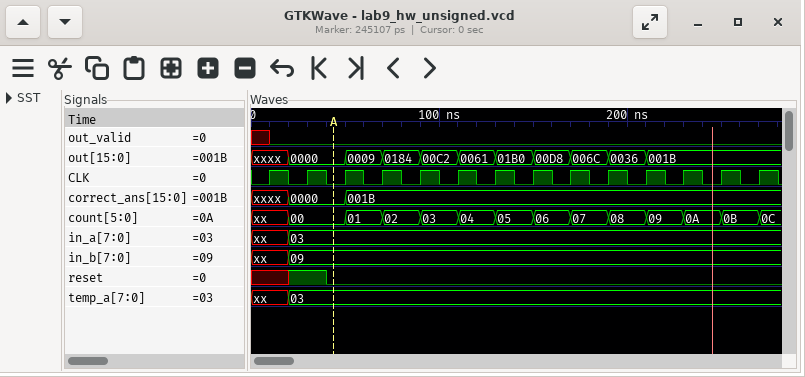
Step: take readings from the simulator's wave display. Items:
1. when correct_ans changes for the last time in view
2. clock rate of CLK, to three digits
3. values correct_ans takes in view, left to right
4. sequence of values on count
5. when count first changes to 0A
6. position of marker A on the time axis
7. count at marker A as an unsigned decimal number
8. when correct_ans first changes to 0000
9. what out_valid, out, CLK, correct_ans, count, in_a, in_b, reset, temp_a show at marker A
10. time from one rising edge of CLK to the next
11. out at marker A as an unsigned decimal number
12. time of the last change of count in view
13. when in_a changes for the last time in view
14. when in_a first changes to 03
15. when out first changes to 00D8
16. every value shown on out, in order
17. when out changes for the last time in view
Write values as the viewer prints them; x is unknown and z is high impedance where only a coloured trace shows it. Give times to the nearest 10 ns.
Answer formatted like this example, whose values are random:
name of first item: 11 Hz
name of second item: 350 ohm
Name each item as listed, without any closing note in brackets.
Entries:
when correct_ans changes for the last time in view: 50 ns
clock rate of CLK, to three digits: 50.0 MHz
values correct_ans takes in view, left to right: xxxx, 0000, 001B
sequence of values on count: xx, 00, 01, 02, 03, 04, 05, 06, 07, 08, 09, 0A, 0B, 0C
when count first changes to 0A: 230 ns
position of marker A on the time axis: 40 ns
count at marker A as an unsigned decimal number: 0
when correct_ans first changes to 0000: 20 ns
what out_valid, out, CLK, correct_ans, count, in_a, in_b, reset, temp_a show at marker A: out_valid=0, out=0000, CLK=0, correct_ans=0000, count=00, in_a=03, in_b=09, reset=0, temp_a=03
time from one rising edge of CLK to the next: 20 ns
out at marker A as an unsigned decimal number: 0
time of the last change of count in view: 270 ns
when in_a changes for the last time in view: 20 ns
when in_a first changes to 03: 20 ns
when out first changes to 00D8: 150 ns
every value shown on out, in order: xxxx, 0000, 0009, 0184, 00C2, 0061, 01B0, 00D8, 006C, 0036, 001B
when out changes for the last time in view: 210 ns
